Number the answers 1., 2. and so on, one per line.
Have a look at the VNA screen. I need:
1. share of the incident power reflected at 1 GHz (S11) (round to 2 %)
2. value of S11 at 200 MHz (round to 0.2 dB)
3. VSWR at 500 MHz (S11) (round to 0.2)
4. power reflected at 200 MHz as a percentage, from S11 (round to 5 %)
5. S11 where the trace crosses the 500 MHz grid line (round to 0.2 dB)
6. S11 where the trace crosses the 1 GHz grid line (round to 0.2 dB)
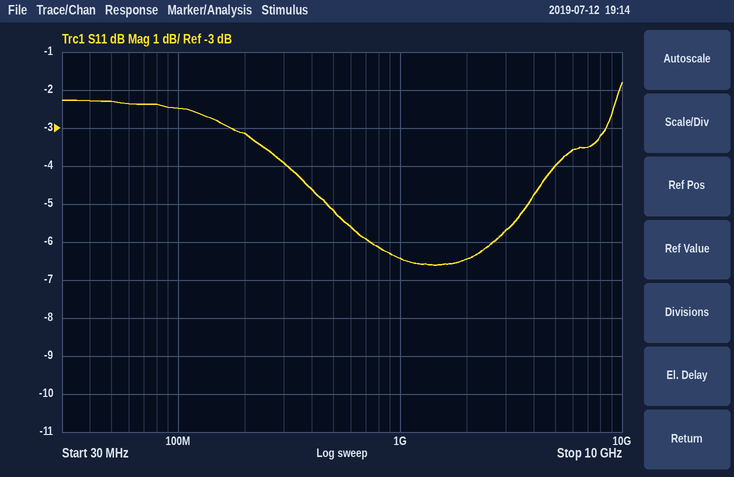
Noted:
1. 22 %
2. -3.2 dB
3. 3.4
4. 50 %
5. -5.2 dB
6. -6.4 dB
